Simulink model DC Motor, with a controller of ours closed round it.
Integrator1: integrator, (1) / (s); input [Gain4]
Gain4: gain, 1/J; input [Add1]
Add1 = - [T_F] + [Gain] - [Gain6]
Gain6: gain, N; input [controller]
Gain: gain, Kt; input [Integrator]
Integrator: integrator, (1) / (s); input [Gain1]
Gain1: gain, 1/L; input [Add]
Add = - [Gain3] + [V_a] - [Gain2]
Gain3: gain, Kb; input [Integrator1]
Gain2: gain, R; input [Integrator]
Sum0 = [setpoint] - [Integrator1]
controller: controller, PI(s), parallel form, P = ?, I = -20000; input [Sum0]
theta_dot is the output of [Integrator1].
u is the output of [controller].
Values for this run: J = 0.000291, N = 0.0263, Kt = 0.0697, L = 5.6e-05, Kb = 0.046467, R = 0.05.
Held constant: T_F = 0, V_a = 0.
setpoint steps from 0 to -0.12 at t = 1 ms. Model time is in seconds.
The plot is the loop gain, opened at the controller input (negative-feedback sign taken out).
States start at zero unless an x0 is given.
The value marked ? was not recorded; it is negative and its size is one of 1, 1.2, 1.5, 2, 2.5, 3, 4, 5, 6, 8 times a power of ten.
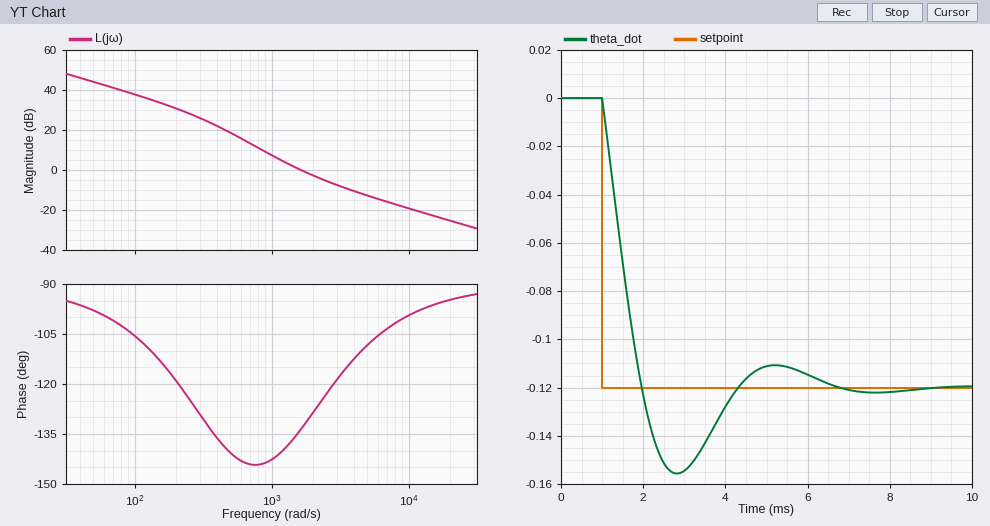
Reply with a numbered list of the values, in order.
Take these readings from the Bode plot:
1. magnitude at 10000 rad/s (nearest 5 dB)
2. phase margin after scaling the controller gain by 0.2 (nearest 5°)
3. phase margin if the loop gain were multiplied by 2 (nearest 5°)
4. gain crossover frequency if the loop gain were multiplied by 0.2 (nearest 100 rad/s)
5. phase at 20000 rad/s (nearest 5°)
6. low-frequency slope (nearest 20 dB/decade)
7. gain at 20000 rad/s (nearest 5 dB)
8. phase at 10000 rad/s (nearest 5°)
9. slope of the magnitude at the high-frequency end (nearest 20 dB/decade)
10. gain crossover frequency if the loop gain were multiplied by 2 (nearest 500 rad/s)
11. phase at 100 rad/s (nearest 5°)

1. -20 dB
2. 35°
3. 60°
4. 700 rad/s
5. -95°
6. -20 dB/decade
7. -25 dB
8. -100°
9. -20 dB/decade
10. 2500 rad/s
11. -105°
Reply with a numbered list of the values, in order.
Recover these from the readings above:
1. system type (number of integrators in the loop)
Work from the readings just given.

1. 1
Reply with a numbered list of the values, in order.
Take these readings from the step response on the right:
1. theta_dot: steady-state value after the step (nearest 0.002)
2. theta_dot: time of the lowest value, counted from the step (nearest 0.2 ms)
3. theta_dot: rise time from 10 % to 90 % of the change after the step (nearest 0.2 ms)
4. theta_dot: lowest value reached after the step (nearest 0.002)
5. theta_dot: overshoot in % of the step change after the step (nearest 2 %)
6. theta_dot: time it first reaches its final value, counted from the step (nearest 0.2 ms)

1. -0.120
2. 1.8 ms
3. 0.8 ms
4. -0.156
5. 30 %
6. 1.0 ms
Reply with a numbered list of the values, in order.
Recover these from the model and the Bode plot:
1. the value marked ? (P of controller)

1. -12
